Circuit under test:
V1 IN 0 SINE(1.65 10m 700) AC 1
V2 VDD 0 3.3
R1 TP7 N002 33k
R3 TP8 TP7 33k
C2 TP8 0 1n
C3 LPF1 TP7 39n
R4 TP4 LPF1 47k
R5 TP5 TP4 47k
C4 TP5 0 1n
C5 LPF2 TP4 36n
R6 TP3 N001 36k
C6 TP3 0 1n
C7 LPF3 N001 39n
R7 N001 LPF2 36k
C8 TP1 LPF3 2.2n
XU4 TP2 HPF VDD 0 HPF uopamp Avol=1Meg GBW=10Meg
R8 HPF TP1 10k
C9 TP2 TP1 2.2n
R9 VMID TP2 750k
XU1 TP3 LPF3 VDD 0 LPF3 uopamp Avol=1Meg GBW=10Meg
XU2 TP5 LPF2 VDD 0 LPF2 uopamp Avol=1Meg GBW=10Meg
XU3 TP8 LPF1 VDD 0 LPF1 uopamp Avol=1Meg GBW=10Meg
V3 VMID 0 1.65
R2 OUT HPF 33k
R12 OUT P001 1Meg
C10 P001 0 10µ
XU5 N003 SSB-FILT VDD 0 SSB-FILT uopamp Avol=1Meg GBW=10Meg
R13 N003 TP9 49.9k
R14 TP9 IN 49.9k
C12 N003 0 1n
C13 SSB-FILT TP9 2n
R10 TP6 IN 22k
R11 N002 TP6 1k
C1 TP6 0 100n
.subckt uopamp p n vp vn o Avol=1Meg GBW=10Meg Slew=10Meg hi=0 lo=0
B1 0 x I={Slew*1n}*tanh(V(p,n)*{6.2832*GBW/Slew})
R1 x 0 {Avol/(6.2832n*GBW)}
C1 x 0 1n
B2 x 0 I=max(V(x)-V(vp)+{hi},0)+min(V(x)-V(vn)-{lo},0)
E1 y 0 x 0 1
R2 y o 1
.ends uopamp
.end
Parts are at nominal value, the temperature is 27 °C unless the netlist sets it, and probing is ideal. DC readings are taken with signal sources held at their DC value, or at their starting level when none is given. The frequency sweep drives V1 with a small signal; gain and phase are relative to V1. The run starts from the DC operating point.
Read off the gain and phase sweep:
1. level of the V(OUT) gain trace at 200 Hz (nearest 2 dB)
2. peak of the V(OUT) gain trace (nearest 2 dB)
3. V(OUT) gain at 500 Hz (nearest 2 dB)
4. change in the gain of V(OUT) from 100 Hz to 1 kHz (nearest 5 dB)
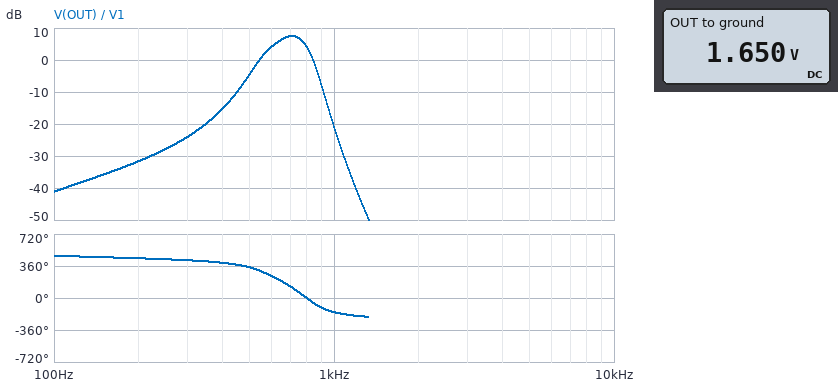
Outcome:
-32 dB
8 dB
-4 dB
20 dB
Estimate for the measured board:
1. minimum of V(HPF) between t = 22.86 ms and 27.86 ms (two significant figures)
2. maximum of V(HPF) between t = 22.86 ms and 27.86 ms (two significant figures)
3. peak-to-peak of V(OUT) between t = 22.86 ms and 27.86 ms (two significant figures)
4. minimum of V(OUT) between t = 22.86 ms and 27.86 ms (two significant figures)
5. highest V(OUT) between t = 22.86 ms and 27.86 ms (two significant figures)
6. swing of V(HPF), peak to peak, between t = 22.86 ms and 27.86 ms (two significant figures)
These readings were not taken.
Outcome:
1.6 V
1.7 V
47 mV
1.6 V
1.7 V
49 mV
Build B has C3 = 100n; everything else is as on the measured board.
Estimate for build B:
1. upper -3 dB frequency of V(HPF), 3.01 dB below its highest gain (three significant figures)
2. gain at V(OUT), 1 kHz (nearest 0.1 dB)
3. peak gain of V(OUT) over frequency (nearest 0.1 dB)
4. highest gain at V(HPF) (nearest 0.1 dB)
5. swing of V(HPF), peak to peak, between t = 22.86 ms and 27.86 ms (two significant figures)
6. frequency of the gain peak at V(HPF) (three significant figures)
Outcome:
661 Hz
-32.8 dB
1.9 dB
2.2 dB
15 mV
546 Hz
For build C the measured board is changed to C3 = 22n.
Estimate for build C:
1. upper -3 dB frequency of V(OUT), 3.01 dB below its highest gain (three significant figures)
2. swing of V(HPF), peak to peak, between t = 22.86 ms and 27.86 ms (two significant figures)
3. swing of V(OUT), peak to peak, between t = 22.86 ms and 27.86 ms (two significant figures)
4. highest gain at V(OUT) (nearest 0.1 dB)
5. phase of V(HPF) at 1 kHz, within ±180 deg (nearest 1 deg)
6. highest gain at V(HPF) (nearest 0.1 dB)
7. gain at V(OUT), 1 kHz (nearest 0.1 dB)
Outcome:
831 Hz
30 mV
29 mV
3.4 dB
-100 deg
3.7 dB
-15.3 dB
